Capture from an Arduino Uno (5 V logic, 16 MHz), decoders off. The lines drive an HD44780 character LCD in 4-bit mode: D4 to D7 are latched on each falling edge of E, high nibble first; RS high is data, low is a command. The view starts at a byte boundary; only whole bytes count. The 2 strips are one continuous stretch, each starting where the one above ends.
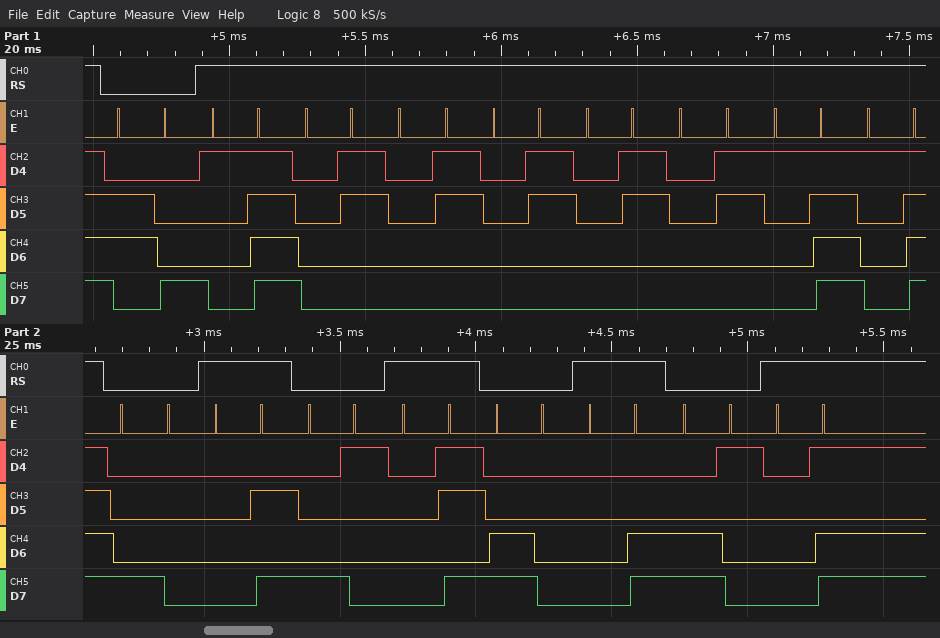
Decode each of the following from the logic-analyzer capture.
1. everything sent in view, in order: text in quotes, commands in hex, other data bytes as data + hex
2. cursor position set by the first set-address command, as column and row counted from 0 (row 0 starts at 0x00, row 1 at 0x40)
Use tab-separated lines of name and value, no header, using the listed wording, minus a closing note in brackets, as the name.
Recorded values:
everything sent in view, in order: text in quotes, commands in hex, other data bytes as data + hex	0x68 data 1F 03 03 03 03 03 1F 1F 0x80 data 0A 0x81 data 0B 0xC0 data 0C 0xC1 data 0D
cursor position set by the first set-address command, as column and row counted from 0	column 0, row 0
